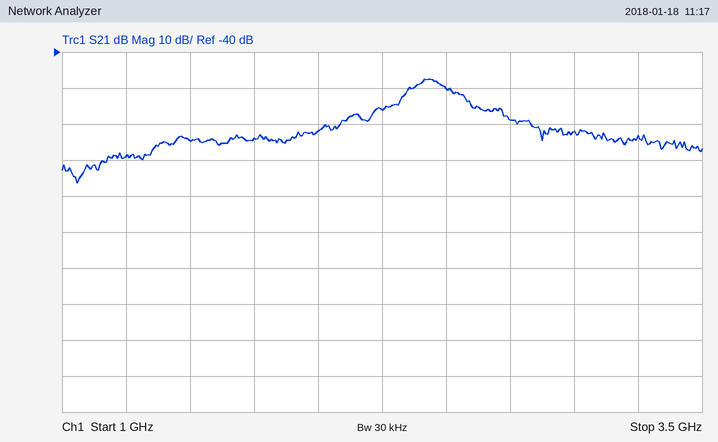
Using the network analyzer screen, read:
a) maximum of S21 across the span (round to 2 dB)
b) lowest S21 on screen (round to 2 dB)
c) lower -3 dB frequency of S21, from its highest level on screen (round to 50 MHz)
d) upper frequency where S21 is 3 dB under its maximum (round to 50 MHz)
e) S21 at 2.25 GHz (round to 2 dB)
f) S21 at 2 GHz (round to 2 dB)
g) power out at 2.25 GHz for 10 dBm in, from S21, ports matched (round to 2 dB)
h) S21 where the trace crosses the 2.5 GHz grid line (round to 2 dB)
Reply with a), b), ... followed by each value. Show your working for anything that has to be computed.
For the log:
a) -48 dB
b) -76 dB
c) 2.35 GHz
d) 2.50 GHz
e) -56 dB
f) -62 dB
g) 10 dBm + (-56 dB) = -46 dBm
h) -50 dB
